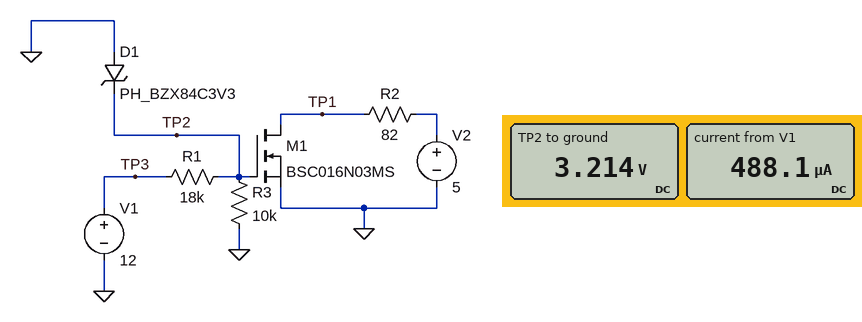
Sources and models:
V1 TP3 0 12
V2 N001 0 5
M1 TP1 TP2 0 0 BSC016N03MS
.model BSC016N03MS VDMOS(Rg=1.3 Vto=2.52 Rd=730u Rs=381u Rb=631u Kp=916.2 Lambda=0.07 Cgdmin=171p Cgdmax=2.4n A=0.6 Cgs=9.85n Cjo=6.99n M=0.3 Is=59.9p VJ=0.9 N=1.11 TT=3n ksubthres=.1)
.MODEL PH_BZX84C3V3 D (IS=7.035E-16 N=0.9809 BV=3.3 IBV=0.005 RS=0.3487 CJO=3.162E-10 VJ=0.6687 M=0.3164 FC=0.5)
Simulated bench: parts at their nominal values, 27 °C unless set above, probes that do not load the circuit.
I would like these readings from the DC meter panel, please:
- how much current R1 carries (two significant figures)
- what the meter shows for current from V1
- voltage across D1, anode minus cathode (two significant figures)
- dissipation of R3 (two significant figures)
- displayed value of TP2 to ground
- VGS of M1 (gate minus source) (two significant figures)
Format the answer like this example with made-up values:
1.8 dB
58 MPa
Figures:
490 µA
488.1 µA
-3.2 V
1.0 mW
3.214 V
3.2 V
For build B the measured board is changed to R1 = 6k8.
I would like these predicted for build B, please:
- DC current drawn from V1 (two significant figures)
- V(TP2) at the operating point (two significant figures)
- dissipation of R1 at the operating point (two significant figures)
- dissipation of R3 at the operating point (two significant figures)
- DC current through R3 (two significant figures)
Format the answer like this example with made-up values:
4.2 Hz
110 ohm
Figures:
1.3 mA
3.3 V
11 mW
1.1 mW
330 µA
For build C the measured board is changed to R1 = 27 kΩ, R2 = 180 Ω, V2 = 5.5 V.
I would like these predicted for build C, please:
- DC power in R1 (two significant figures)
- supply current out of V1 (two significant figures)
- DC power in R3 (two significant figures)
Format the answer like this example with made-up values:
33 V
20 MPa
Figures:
2.9 mW
330 µA
990 µW
